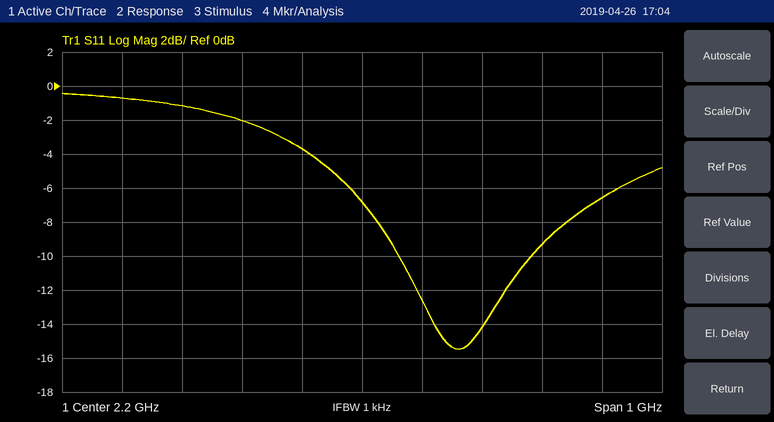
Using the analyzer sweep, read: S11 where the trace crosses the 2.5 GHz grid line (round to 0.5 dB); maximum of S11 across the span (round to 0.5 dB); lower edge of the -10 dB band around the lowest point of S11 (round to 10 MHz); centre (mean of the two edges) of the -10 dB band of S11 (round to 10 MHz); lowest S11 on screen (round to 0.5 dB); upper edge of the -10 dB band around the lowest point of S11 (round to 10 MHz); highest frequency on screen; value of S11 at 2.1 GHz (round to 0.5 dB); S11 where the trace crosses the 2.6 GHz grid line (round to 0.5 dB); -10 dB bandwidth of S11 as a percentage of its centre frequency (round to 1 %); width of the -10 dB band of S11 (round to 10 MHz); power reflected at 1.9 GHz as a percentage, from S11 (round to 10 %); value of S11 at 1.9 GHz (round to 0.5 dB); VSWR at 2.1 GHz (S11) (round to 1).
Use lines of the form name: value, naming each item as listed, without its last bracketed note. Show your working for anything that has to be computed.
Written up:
S11 where the trace crosses the 2.5 GHz grid line: -9.5 dB
maximum of S11 across the span: -0.5 dB
lower edge of the -10 dB band around the lowest point of S11: 2.26 GHz
centre (mean of the two edges) of the -10 dB band of S11: 2.37 GHz
lowest S11 on screen: -15.5 dB
upper edge of the -10 dB band around the lowest point of S11: 2.48 GHz
highest frequency on screen: 2.7 GHz
value of S11 at 2.1 GHz: -3.5 dB
S11 where the trace crosses the 2.6 GHz grid line: -6.5 dB
-10 dB bandwidth of S11 as a percentage of its centre frequency: 220 MHz / 2.37 GHz ≈ 9 %
width of the -10 dB band of S11: 2.48 GHz − 2.26 GHz = 220 MHz
power reflected at 1.9 GHz as a percentage, from S11: 10^(-1/10) ≈ 79.4 %, so 80 % to the nearest 10 %
value of S11 at 1.9 GHz: -1.0 dB
VSWR at 2.1 GHz (S11): |Γ| = 10^(-3.5/20) = 0.6683; VSWR = (1 + 0.6683)/(1 − 0.6683) ≈ 5
